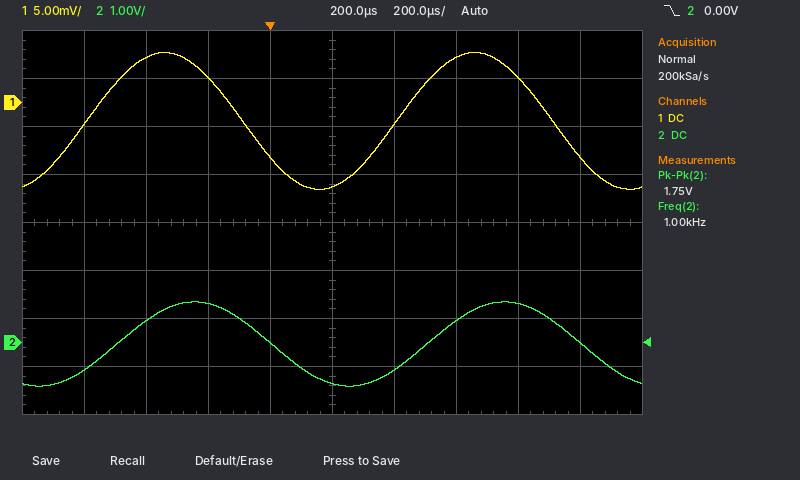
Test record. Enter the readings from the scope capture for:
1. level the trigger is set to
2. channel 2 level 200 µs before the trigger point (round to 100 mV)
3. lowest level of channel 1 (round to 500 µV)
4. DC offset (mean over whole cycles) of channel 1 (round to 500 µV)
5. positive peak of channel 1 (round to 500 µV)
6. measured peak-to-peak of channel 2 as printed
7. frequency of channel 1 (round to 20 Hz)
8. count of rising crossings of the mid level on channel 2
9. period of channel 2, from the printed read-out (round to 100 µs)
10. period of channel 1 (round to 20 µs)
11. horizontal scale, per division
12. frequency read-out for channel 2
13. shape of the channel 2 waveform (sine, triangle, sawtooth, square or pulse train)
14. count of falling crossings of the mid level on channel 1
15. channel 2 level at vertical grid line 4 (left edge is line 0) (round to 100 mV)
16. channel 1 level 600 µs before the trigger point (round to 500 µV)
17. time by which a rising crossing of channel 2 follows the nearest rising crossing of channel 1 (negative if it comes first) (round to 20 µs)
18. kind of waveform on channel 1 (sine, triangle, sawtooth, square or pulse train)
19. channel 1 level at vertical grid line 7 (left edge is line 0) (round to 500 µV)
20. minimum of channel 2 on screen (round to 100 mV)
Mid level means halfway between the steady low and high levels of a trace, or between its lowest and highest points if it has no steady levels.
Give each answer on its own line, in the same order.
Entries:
0.00 V
800 mV
-9.0 mV
-2.0 mV
5.0 mV
1.75 V
1.00 kHz
2
1.0 ms
1.00 ms
200 µs
1.00 kHz
sine
2
0.0 V
-2.5 mV
+100 µs
sine
4.5 mV
-900 mV
